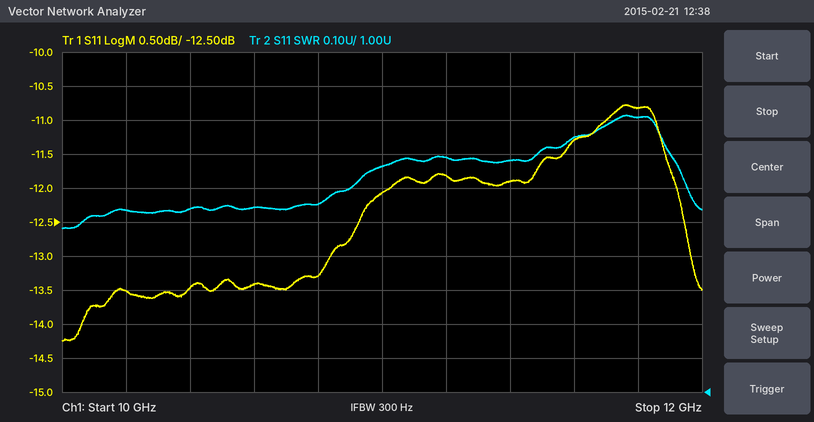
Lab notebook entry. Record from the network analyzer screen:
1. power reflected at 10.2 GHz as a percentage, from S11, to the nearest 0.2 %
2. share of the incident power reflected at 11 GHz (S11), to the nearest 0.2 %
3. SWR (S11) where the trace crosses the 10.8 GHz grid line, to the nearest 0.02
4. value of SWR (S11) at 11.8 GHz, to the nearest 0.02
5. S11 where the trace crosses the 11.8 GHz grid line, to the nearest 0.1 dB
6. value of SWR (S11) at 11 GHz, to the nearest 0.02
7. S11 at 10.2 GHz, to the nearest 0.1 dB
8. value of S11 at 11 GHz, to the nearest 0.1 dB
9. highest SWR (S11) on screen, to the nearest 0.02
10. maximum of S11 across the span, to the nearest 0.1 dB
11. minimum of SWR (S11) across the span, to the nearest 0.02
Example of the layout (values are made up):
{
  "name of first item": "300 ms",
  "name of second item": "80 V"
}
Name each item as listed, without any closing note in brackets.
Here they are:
{
  "power reflected at 10.2 GHz as a percentage, from S11, to the nearest 0.2 %": "4.4 %",
  "share of the incident power reflected at 11 GHz (S11), to the nearest 0.2 %": "6.2 %",
  "SWR (S11) where the trace crosses the 10.8 GHz grid line, to the nearest 0.02": "1.56",
  "value of SWR (S11) at 11.8 GHz, to the nearest 0.02": "1.80",
  "S11 where the trace crosses the 11.8 GHz grid line, to the nearest 0.1 dB": "-10.8 dB",
  "value of SWR (S11) at 11 GHz, to the nearest 0.02": "1.66",
  "S11 at 10.2 GHz, to the nearest 0.1 dB": "-13.5 dB",
  "value of S11 at 11 GHz, to the nearest 0.1 dB": "-12.1 dB",
  "highest SWR (S11) on screen, to the nearest 0.02": "1.82",
  "maximum of S11 across the span, to the nearest 0.1 dB": "-10.8 dB",
  "minimum of SWR (S11) across the span, to the nearest 0.02": "1.48"
}
